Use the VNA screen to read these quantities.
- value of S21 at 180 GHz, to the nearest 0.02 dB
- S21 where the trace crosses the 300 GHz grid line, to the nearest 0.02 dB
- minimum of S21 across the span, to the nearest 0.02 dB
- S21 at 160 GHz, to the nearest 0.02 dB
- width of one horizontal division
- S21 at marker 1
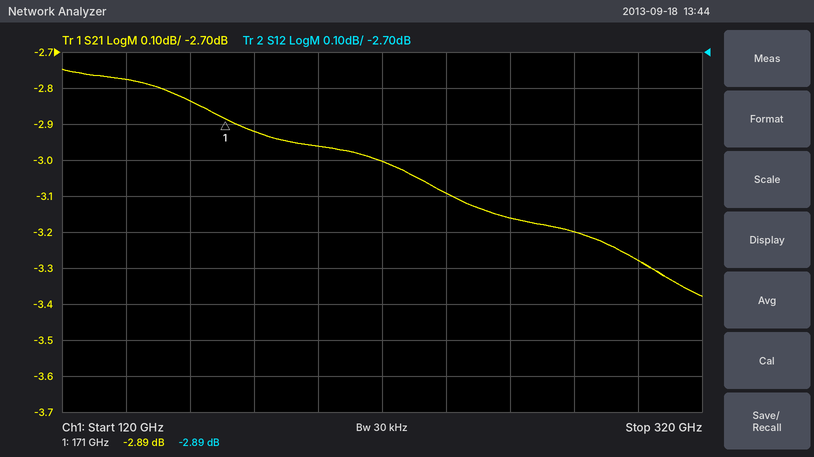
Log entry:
-2.92 dB
-3.28 dB
-3.38 dB
-2.84 dB
20 GHz
-2.89 dB
